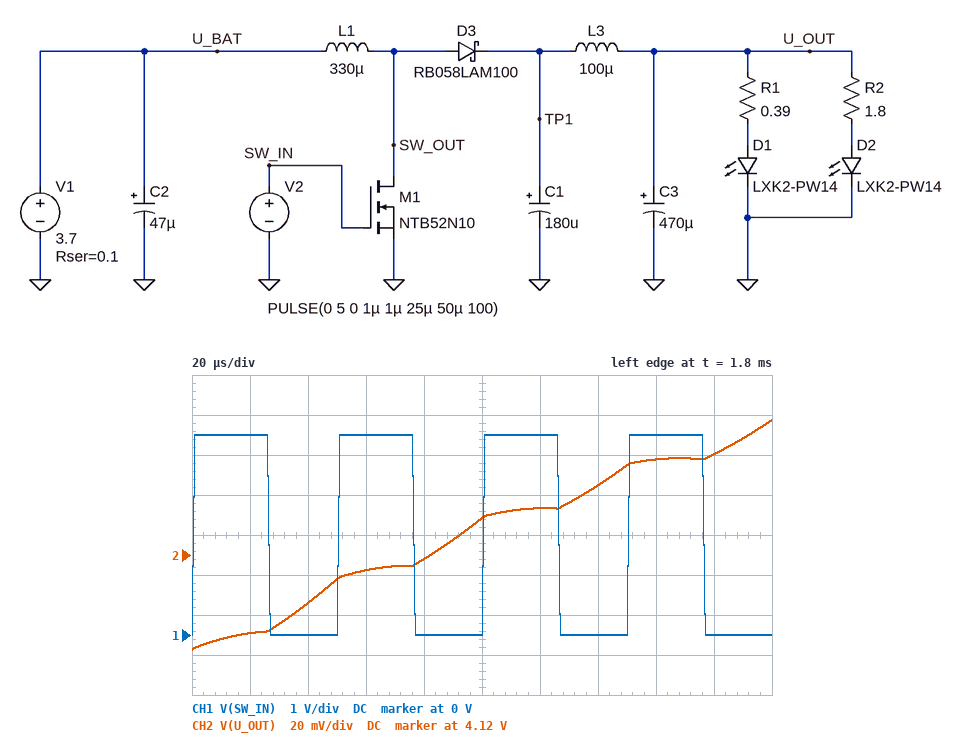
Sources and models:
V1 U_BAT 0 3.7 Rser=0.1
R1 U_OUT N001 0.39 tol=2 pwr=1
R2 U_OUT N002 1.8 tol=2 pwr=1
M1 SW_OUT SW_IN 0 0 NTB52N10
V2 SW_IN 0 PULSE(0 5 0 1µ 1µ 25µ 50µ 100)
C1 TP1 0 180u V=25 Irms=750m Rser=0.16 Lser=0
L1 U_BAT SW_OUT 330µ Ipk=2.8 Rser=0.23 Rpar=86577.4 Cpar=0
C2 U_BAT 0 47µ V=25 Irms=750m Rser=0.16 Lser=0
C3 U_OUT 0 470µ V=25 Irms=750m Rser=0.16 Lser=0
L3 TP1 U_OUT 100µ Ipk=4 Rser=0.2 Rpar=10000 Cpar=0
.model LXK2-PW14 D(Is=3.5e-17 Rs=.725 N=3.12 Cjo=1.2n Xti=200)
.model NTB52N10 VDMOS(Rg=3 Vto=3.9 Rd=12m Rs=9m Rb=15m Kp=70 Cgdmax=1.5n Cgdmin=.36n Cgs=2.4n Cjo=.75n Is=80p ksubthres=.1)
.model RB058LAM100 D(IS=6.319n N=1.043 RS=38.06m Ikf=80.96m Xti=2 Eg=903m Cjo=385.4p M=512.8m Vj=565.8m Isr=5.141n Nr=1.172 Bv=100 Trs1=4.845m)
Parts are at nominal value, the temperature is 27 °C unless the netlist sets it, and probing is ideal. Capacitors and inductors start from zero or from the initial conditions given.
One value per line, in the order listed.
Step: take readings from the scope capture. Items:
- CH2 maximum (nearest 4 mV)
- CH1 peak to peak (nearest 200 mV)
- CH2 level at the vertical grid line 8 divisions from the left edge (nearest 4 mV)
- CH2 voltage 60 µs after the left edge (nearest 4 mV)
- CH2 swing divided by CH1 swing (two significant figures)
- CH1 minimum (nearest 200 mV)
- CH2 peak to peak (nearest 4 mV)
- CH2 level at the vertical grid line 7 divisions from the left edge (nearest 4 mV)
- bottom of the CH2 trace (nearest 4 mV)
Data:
4.188 V
5.0 V
4.168 V
4.112 V
0.023
0 V
116 mV
4.156 V
4.072 V
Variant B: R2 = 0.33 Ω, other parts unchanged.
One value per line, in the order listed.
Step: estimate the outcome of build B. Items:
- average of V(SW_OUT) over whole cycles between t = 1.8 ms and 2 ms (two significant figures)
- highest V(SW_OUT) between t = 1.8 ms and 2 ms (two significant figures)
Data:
2.7 V
5.5 V
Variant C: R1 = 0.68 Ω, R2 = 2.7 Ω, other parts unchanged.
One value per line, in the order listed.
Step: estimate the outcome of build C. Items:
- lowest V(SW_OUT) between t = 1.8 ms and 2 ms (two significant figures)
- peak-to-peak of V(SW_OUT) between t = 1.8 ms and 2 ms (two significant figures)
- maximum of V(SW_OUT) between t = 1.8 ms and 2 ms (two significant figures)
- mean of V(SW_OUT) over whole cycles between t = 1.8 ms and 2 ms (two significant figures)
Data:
120 mV
5.7 V
5.8 V
2.9 V
